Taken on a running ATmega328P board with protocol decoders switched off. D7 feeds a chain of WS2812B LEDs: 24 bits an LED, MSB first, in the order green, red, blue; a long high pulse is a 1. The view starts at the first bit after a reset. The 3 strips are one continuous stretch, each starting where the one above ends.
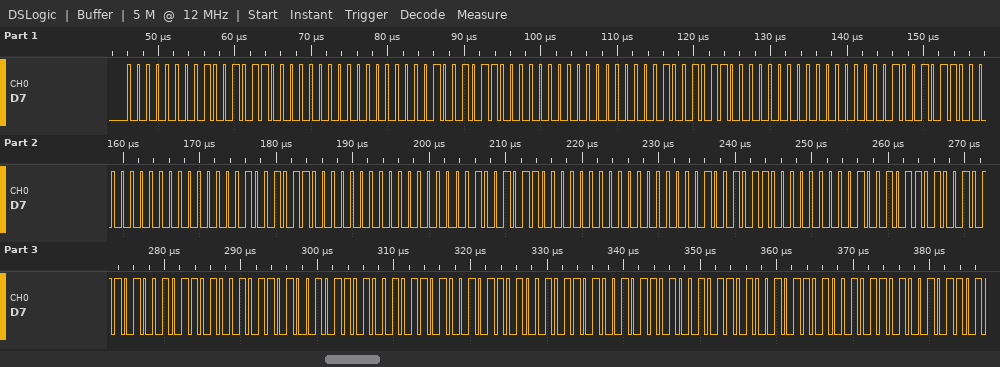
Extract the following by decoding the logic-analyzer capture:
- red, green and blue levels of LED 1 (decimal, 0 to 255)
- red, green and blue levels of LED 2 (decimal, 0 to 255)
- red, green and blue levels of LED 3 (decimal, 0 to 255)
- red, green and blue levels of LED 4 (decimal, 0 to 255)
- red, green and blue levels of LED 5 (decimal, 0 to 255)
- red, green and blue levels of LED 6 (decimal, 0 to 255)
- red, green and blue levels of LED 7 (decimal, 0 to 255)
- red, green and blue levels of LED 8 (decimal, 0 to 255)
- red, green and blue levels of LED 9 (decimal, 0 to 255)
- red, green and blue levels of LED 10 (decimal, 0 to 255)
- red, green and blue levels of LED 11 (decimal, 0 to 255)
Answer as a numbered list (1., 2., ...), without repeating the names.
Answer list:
1. 150, 0, 0
2. 150, 0, 0
3. 150, 0, 0
4. 150, 0, 0
5. 150, 0, 0
6. 150, 0, 0
7. 150, 0, 0
8. 150, 150, 150
9. 150, 150, 150
10. 150, 150, 150
11. 150, 150, 150
